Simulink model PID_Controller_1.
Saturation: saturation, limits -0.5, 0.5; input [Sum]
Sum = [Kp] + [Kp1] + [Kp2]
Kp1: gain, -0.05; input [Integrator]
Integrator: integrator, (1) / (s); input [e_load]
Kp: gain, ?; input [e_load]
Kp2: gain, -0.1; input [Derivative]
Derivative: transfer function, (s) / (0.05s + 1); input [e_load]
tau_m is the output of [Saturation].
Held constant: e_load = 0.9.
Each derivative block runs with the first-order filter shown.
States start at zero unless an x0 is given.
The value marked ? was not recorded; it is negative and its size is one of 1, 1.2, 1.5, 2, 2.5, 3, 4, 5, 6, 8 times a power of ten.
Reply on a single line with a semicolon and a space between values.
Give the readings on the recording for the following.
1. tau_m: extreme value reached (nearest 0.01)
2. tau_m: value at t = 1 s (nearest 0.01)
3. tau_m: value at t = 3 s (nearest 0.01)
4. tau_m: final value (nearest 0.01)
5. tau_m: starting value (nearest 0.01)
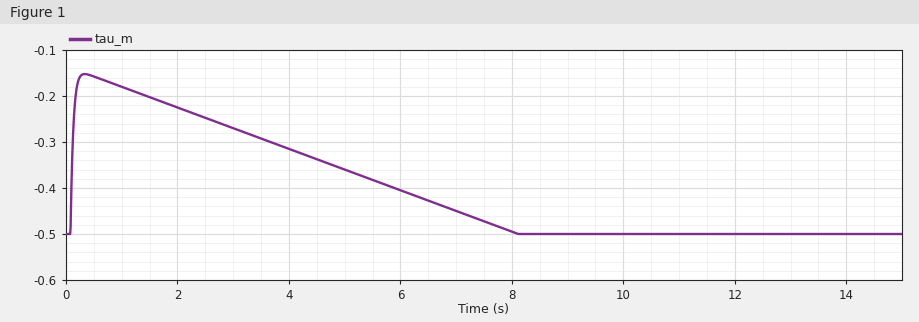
-0.15; -0.18; -0.27; -0.50; -0.50
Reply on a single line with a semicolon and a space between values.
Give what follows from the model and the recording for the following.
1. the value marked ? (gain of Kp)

-0.15
